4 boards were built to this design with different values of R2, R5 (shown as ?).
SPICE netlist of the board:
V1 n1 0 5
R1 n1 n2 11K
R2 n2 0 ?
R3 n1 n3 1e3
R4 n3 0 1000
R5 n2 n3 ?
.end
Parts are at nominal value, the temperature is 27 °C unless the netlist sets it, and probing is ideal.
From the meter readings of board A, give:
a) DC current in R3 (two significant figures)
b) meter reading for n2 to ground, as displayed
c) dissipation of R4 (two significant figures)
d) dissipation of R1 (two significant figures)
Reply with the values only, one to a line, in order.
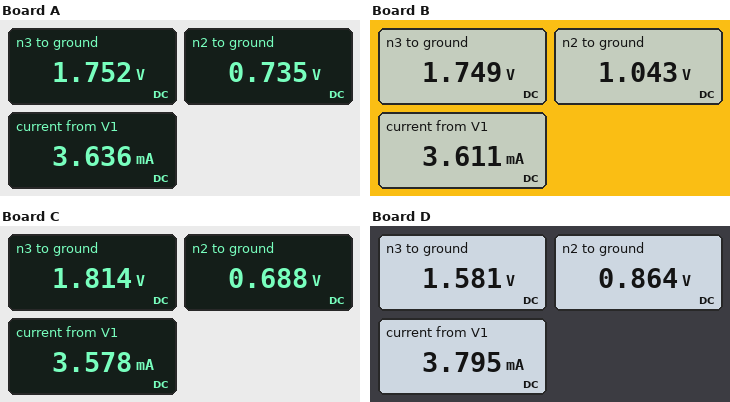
3.2 mA
0.735 V
3.1 mW
1.7 mW
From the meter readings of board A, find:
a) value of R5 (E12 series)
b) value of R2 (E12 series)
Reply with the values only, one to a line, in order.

680 Ω
390 Ω
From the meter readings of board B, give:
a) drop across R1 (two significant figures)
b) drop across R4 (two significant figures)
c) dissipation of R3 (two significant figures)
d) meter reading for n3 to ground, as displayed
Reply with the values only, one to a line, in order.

4.0 V
1.7 V
11 mW
1.749 V
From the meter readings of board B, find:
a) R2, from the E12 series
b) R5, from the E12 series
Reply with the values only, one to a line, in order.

560 Ω
470 Ω
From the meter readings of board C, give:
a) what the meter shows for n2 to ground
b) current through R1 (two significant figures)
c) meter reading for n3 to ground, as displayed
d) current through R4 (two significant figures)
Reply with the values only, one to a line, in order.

0.688 V
390 µA
1.814 V
1.8 mA
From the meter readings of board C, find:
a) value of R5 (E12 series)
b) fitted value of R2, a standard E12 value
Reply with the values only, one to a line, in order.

820 Ω
390 Ω
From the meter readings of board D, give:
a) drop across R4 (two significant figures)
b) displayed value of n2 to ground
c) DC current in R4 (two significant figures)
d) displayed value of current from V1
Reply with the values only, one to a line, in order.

1.6 V
0.864 V
1.6 mA
3.795 mA
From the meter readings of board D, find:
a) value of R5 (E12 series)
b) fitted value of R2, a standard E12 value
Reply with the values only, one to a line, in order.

390 Ω
390 Ω
